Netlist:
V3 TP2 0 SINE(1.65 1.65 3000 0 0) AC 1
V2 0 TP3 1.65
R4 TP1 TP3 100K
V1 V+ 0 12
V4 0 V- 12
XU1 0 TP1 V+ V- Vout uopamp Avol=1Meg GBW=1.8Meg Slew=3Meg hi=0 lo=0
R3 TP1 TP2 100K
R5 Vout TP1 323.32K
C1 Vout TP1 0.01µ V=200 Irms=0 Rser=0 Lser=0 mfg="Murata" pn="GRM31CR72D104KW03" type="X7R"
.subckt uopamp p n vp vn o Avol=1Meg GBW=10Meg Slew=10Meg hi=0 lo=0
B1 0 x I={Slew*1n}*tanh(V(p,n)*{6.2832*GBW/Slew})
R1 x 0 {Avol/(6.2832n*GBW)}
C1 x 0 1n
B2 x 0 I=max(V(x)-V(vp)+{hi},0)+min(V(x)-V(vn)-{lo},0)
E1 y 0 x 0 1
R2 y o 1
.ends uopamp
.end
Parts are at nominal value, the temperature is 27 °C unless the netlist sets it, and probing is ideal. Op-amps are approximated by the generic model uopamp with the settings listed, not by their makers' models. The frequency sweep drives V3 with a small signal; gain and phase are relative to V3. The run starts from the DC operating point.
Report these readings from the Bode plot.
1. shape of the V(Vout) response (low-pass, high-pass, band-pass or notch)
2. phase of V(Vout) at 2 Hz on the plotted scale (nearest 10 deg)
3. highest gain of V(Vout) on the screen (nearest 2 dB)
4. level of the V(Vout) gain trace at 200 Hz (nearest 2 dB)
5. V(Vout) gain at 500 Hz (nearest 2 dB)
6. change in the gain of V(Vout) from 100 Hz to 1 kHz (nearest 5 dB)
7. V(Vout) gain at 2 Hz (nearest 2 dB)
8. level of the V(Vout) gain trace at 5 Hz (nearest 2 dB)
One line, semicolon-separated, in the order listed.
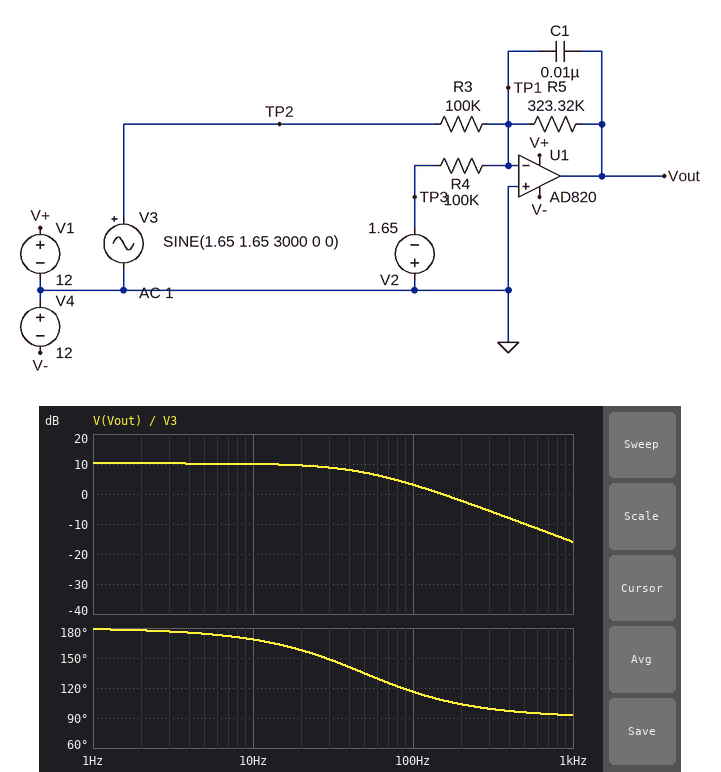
low-pass; 180 deg; 10 dB; -2 dB; -10 dB; -20 dB; 10 dB; 10 dB
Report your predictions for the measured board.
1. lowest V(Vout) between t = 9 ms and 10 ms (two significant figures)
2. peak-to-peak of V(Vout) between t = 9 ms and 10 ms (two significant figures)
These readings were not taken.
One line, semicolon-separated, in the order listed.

-93 mV; 180 mV
